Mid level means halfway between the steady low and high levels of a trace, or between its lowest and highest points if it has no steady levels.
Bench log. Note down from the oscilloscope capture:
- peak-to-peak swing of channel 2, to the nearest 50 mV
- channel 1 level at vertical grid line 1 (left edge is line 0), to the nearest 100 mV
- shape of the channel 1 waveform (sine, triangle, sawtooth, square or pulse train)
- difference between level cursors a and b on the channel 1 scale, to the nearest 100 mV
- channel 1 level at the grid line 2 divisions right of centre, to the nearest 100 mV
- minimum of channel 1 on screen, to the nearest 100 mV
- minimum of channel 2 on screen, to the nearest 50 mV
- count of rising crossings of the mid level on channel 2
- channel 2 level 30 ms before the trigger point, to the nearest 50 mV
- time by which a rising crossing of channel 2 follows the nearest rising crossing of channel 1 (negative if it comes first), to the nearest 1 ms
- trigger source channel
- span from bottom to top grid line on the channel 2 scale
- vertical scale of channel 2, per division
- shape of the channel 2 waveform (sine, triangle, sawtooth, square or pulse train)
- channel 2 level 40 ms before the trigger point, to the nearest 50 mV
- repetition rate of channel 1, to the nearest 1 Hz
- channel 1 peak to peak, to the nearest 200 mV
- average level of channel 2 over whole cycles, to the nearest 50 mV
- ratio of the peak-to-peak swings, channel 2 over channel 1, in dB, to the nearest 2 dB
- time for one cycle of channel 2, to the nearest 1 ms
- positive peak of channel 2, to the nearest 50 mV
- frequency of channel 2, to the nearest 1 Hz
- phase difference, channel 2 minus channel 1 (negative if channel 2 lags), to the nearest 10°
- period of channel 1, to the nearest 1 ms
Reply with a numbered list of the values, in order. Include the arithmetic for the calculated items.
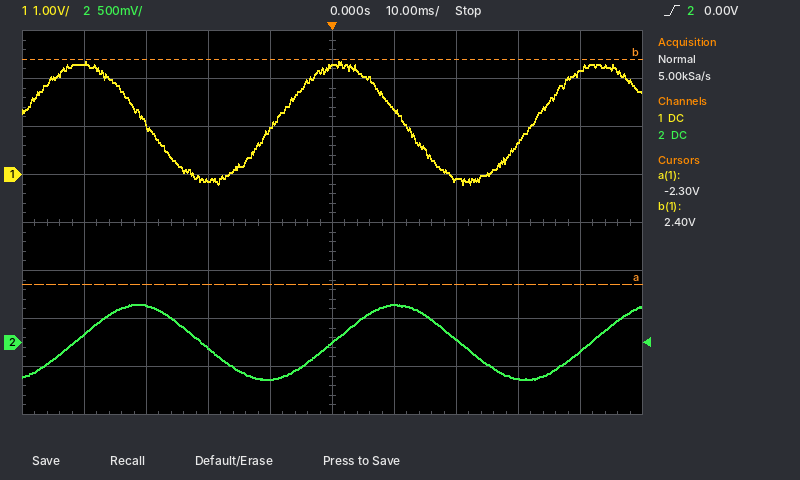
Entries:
1. 400 mV − (-400 mV) = 800 mV
2. 2.3 V
3. sine
4. 4.7 V
5. -100 mV
6. -200 mV
7. -400 mV
8. 3
9. 400 mV
10. +9 ms
11. channel 2
12. 4 V
13. 500 mV
14. sine
15. 100 mV
16. 1 / 42 ms ≈ 24 Hz
17. 2.6 V
18. (400 mV + (-400 mV)) / 2 ≈ 0 mV
19. 20 log10(800 mV / 2.6 V) ≈ -10 dB
20. 42 ms
21. 400 mV
22. 1 / 42 ms ≈ 24 Hz
23. −360° × (+9 ms) / 42 ms ≈ -77.1°, so -80° to the nearest 10°
24. 42 ms
